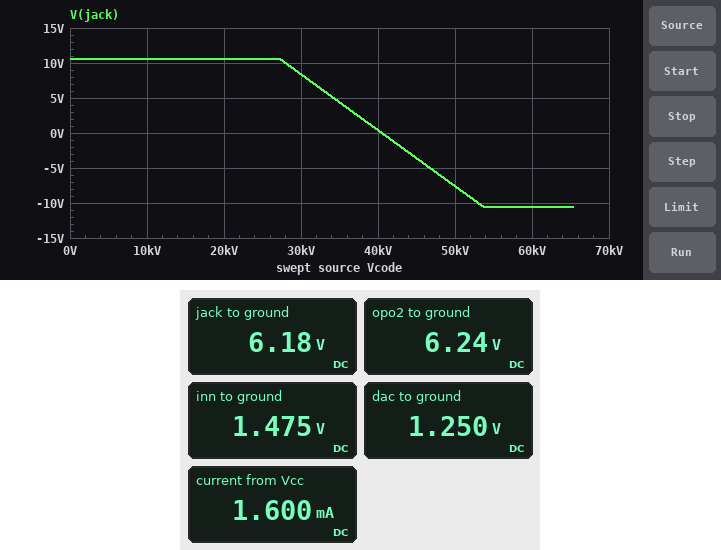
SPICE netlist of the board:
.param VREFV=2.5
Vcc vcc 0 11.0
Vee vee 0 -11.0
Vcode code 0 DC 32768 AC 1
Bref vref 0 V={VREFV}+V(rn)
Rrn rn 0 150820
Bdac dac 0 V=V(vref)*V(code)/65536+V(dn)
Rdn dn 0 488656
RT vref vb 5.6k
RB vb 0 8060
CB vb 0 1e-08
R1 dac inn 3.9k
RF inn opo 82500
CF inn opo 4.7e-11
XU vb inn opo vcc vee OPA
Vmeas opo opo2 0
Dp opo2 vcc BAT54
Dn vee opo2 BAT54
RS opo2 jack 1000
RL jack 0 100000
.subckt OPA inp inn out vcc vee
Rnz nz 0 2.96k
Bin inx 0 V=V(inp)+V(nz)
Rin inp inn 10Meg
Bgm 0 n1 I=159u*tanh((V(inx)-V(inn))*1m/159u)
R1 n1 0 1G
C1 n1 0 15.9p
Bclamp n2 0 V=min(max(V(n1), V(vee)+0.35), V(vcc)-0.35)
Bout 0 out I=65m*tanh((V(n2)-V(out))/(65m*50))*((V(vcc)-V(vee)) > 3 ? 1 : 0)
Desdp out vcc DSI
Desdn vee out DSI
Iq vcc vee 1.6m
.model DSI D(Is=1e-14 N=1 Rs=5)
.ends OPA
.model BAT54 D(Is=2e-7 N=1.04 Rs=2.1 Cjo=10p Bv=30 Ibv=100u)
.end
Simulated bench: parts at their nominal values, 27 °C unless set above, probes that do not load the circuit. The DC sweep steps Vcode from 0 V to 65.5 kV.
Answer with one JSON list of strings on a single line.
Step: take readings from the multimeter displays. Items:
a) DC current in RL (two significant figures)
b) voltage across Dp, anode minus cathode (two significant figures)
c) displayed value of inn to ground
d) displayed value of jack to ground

["62 µA", "-4.8 V", "1.475 V", "6.18 V"]
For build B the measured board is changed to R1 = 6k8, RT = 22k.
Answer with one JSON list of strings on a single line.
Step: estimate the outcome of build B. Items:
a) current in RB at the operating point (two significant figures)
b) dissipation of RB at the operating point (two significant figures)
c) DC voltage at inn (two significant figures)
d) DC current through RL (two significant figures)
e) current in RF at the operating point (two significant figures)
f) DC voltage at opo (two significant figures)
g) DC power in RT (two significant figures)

["83 µA", "56 µW", "670 mV", "63 µA", "85 µA", "-6.4 V", "150 µW"]
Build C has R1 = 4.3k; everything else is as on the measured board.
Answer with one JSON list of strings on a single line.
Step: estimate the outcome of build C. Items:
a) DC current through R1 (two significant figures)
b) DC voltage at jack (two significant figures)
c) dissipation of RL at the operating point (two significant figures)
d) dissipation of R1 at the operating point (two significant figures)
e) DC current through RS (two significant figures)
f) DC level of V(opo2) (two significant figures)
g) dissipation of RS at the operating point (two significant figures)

["52 µA", "5.7 V", "330 µW", "12 µW", "57 µA", "5.8 V", "3.3 µW"]
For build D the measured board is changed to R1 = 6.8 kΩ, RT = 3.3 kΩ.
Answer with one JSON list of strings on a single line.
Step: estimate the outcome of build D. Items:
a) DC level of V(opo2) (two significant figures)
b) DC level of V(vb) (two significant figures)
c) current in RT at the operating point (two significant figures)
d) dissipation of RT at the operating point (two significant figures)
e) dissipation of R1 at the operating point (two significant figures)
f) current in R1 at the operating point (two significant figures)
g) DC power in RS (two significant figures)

["8.1 V", "1.8 V", "220 µA", "160 µW", "40 µW", "77 µA", "6.5 µW"]
